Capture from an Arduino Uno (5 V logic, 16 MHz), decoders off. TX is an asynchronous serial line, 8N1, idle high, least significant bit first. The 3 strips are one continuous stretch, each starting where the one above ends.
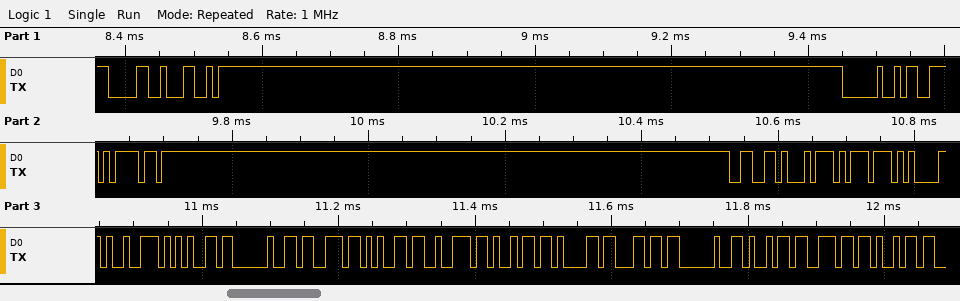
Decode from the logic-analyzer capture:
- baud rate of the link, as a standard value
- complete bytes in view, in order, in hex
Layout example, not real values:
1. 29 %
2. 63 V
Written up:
1. 115200 baud
2. 30 4C 20 73 6F 66 74 77 61 72 65 20 73 65 72 69 61 6C 20 69 6E 69
